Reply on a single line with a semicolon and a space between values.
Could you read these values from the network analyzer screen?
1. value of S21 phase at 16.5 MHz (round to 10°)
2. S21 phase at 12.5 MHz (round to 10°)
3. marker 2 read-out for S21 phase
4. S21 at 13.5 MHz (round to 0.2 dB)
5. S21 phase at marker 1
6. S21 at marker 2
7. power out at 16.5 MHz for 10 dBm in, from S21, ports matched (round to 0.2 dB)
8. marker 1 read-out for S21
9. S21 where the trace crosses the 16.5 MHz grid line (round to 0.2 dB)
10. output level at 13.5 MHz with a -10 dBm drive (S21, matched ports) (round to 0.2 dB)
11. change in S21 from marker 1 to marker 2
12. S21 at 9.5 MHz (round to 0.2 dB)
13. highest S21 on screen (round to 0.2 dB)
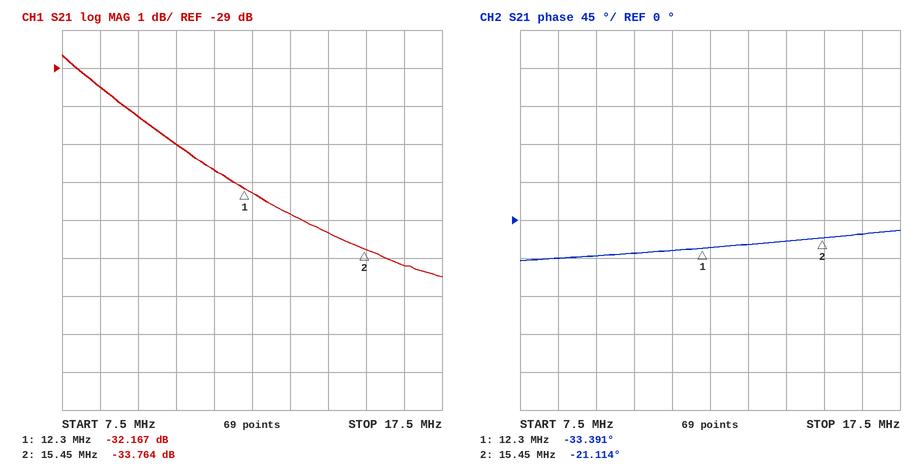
-20°; -30°; -21.114°; -32.8 dB; -33.391°; -33.764 dB; -24.2 dBm; -32.167 dB; -34.2 dB; -42.8 dBm; -1.597 dB; -30.2 dB; -28.6 dB
